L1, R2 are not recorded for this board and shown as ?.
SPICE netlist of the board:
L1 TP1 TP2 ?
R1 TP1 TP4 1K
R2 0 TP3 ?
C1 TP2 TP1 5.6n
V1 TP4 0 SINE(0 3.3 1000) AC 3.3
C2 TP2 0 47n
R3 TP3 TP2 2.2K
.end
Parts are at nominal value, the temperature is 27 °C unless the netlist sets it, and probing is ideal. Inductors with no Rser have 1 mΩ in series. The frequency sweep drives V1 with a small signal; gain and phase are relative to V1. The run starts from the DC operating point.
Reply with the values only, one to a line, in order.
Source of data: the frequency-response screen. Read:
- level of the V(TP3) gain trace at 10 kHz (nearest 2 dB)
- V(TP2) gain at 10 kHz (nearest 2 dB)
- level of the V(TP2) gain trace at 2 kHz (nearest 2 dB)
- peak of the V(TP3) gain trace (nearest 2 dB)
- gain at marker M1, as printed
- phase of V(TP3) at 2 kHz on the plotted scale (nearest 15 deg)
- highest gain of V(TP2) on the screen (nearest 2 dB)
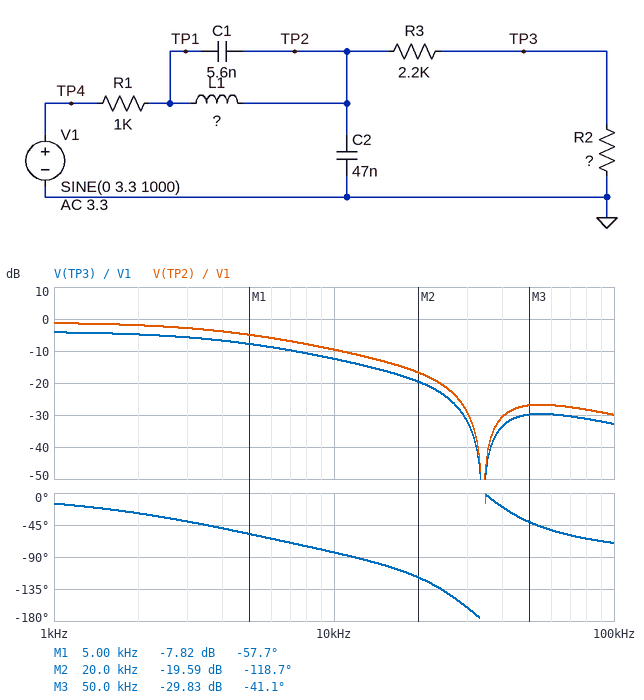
-12 dB
-10 dB
-2 dB
-4 dB
-7.82 dB
-30 deg
-2 dB
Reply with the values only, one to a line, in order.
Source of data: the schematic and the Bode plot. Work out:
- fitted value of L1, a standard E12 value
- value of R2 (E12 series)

3.9 mH
5.6 kΩ
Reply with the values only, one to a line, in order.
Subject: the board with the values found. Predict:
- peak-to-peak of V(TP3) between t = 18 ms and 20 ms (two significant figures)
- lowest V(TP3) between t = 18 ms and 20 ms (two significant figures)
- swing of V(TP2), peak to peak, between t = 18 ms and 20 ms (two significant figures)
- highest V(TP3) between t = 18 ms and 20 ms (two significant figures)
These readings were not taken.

4.1 V
-2.0 V
5.7 V
2.0 V
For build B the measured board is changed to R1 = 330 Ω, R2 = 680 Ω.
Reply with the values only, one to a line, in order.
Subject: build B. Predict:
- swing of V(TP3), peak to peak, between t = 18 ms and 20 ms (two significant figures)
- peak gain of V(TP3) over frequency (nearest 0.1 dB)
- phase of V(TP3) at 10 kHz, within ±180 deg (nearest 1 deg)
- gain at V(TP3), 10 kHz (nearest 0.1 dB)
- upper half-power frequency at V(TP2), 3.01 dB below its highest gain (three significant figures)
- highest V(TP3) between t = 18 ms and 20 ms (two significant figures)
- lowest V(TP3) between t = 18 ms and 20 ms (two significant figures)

1.4 V
-13.0 dB
-73 deg
-13.5 dB
13.3 kHz
700 mV
-700 mV
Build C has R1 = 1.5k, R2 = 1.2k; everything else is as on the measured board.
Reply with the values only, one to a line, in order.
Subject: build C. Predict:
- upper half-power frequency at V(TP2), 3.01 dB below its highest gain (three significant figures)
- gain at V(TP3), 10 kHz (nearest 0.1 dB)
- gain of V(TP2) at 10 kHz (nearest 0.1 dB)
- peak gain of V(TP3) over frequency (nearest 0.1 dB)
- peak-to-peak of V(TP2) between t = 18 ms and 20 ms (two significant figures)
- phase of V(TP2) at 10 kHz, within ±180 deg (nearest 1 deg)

3.38 kHz
-22.2 dB
-13.2 dB
-12.2 dB
4.4 V
-82 deg
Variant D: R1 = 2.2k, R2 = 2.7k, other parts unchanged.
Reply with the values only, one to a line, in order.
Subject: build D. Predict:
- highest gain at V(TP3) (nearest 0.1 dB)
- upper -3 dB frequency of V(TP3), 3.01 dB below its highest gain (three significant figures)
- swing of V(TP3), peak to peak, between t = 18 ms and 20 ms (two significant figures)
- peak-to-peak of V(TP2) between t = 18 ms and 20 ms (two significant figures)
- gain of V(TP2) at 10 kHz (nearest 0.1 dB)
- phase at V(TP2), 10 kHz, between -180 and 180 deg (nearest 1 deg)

-8.4 dB
2.27 kHz
2.3 V
4.2 V
-16.4 dB
-84 deg
